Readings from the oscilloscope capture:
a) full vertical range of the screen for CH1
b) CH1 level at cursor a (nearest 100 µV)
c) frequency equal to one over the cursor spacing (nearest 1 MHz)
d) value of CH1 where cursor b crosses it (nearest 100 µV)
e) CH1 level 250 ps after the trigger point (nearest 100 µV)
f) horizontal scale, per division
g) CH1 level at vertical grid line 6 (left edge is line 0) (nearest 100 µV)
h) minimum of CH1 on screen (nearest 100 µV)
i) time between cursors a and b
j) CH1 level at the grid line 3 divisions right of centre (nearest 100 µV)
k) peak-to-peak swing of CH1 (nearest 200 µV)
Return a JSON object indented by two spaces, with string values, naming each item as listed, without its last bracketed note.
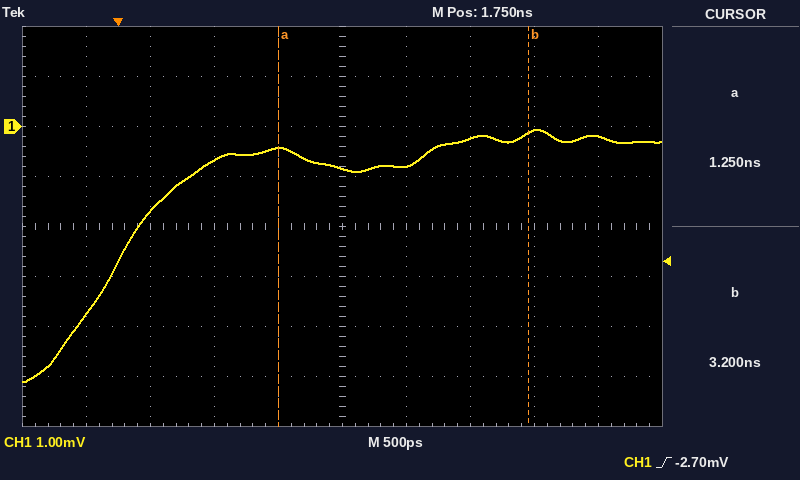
{
  "full vertical range of the screen for CH1": "8 mV",
  "CH1 level at cursor a": "-400 µV",
  "frequency equal to one over the cursor spacing": "513 MHz",
  "value of CH1 where cursor b crosses it": "-100 µV",
  "CH1 level 250 ps after the trigger point": "-1.7 mV",
  "horizontal scale, per division": "500 ps",
  "CH1 level at vertical grid line 6 (left edge is line 0)": "-800 µV",
  "minimum of CH1 on screen": "-5.1 mV",
  "time between cursors a and b": "1.95 ns",
  "CH1 level at the grid line 3 divisions right of centre": "-100 µV",
  "peak-to-peak swing of CH1": "5.0 mV"
}
